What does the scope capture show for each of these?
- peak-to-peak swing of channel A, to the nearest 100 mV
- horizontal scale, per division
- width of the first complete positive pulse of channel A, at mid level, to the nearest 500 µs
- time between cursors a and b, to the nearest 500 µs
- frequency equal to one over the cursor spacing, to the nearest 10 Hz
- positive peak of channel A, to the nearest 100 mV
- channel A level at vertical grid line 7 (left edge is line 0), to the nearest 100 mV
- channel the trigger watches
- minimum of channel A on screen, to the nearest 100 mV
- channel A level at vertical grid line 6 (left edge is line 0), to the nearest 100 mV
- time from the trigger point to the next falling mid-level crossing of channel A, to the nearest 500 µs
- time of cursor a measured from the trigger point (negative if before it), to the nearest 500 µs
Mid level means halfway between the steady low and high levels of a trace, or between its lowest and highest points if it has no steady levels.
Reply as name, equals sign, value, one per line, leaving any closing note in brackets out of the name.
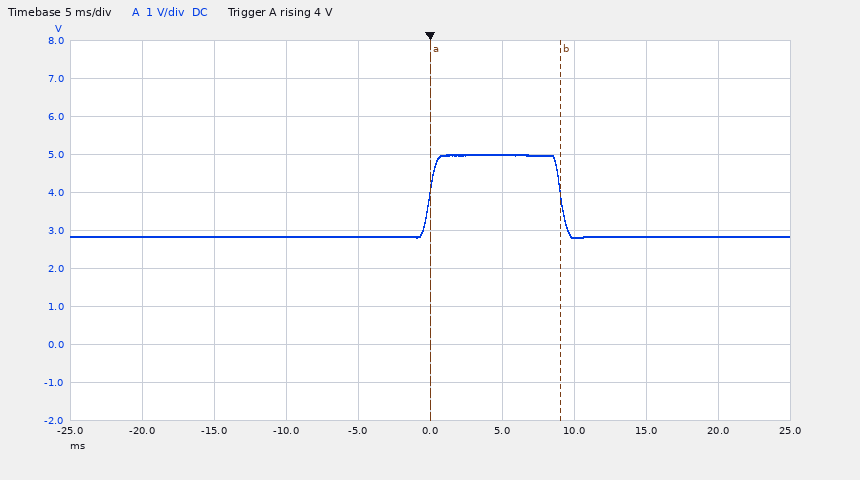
peak-to-peak swing of channel A, to the nearest 100 mV = 2.2 V
horizontal scale, per division = 5 ms
width of the first complete positive pulse of channel A, at mid level, to the nearest 500 µs = 9.0 ms
time between cursors a and b, to the nearest 500 µs = 9.0 ms
frequency equal to one over the cursor spacing, to the nearest 10 Hz = 110 Hz
positive peak of channel A, to the nearest 100 mV = 5.0 V
channel A level at vertical grid line 7 (left edge is line 0), to the nearest 100 mV = 2.8 V
channel the trigger watches = channel A
minimum of channel A on screen, to the nearest 100 mV = 2.8 V
channel A level at vertical grid line 6 (left edge is line 0), to the nearest 100 mV = 5.0 V
time from the trigger point to the next falling mid-level crossing of channel A, to the nearest 500 µs = 9.0 ms
time of cursor a measured from the trigger point (negative if before it), to the nearest 500 µs = 0.0 ms
